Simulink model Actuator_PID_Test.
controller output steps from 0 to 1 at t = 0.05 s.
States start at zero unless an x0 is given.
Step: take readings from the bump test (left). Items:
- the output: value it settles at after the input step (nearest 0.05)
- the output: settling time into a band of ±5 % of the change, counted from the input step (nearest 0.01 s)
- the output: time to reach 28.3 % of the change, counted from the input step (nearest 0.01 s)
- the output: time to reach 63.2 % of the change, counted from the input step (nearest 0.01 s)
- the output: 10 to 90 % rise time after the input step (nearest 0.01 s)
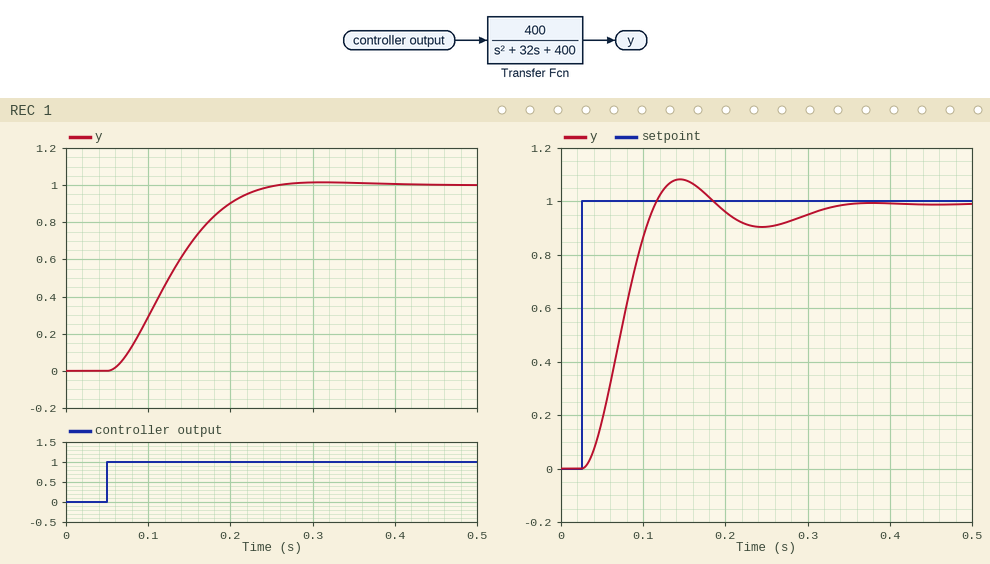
1.00
0.17 s
0.05 s
0.09 s
0.12 s
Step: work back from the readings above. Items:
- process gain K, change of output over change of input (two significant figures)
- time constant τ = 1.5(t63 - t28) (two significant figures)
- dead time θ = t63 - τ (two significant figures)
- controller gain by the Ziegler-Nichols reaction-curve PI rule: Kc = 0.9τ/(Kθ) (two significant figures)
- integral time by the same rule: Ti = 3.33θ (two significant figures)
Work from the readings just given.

1.0
0.060 s
0.030 s
1.8
0.100 s
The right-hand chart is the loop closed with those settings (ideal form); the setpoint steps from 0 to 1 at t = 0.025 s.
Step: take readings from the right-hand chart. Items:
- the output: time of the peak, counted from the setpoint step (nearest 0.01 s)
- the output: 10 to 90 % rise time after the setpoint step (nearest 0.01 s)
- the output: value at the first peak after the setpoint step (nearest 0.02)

0.12 s
0.06 s
1.08
